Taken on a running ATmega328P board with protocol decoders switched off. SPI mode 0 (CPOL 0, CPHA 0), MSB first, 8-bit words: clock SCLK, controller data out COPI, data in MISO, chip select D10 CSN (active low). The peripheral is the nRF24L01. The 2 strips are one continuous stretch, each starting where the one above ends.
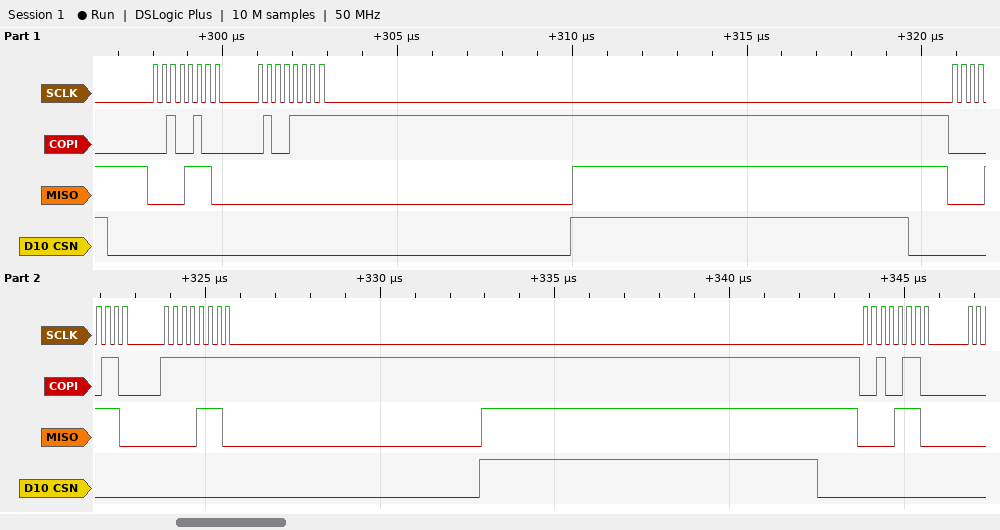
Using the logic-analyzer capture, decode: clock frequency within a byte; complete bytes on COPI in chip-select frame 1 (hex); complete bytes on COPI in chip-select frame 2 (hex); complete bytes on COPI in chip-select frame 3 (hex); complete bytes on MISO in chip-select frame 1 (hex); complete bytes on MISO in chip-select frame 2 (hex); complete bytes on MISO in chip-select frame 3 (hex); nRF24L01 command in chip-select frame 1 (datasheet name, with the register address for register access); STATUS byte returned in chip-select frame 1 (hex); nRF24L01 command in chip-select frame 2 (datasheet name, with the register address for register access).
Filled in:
4 MHz
24 4F
06 FF
26
0E 00
0E 0E
0E
W_REGISTER 0x04
0x0E
R_REGISTER 0x06
